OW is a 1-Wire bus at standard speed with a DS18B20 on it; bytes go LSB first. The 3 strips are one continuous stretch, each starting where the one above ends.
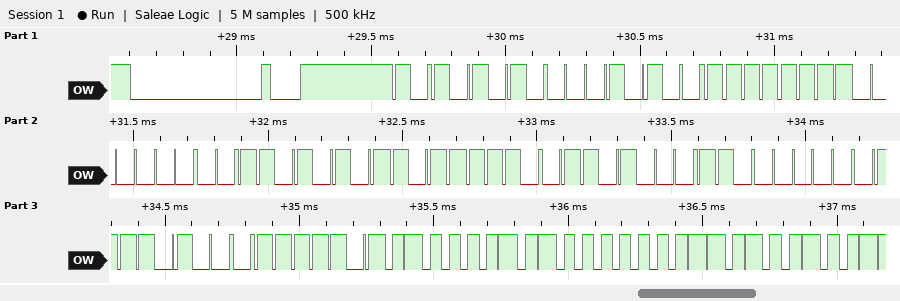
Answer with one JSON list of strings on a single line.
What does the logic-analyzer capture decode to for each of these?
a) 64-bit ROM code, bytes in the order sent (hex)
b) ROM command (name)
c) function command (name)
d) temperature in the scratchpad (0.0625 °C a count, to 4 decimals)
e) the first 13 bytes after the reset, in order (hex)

["28 FF 00 AB 7D 16 03 2E", "Match ROM", "Read Scratchpad", "20.1250 °C", "55 28 FF 00 AB 7D 16 03 2E BE 42 01 4B"]
